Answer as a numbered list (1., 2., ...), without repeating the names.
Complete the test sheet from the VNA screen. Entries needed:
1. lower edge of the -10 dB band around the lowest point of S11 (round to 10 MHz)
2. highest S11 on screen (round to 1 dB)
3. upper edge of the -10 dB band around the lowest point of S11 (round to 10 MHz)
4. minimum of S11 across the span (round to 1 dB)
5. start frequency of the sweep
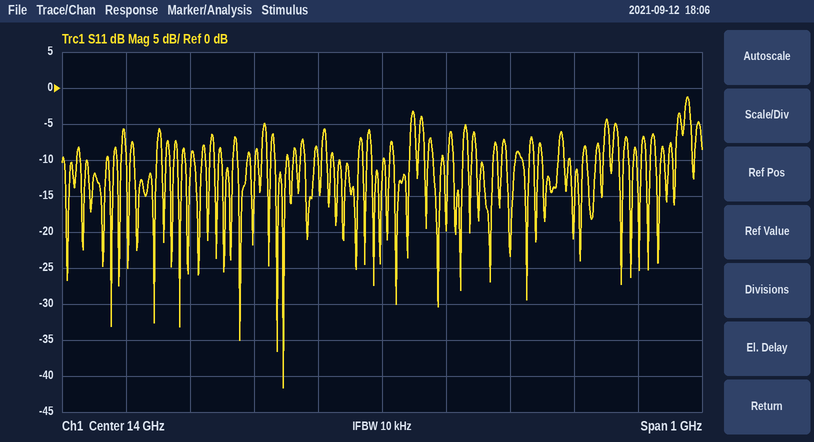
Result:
1. 13.83 GHz
2. -1 dB
3. 13.85 GHz
4. -42 dB
5. 13.5 GHz
